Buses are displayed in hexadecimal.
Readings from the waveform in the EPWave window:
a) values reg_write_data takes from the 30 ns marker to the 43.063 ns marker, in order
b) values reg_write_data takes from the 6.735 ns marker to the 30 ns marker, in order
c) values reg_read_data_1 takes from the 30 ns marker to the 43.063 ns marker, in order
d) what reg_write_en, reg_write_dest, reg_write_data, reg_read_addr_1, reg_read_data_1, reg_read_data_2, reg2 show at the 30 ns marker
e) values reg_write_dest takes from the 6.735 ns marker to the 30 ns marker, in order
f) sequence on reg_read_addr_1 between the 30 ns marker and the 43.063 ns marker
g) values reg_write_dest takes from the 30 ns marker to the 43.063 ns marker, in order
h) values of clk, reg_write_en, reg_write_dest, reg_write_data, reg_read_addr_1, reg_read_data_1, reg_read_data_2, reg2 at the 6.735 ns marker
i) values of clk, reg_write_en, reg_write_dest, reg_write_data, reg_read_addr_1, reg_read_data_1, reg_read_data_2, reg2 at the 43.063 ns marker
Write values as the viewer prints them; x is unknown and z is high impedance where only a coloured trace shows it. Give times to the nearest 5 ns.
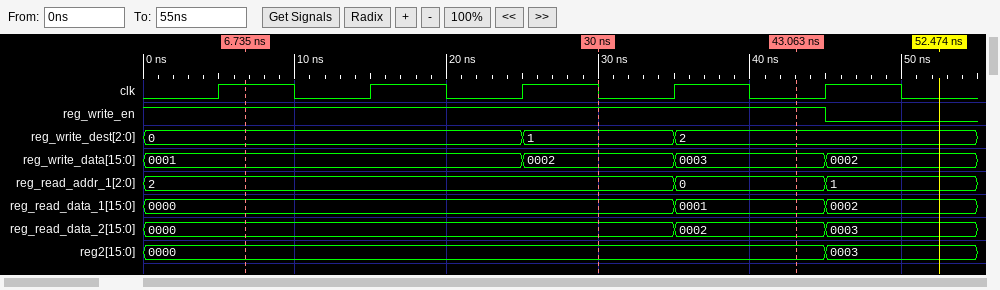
0002, 0003
0001, 0002
0000, 0001
reg_write_en=1, reg_write_dest=1, reg_write_data=0002, reg_read_addr_1=2, reg_read_data_1=0000, reg_read_data_2=0000, reg2=0000
0, 1
2, 0
1, 2
clk=1, reg_write_en=1, reg_write_dest=0, reg_write_data=0001, reg_read_addr_1=2, reg_read_data_1=0000, reg_read_data_2=0000, reg2=0000
clk=0, reg_write_en=1, reg_write_dest=2, reg_write_data=0003, reg_read_addr_1=0, reg_read_data_1=0001, reg_read_data_2=0002, reg2=0000
